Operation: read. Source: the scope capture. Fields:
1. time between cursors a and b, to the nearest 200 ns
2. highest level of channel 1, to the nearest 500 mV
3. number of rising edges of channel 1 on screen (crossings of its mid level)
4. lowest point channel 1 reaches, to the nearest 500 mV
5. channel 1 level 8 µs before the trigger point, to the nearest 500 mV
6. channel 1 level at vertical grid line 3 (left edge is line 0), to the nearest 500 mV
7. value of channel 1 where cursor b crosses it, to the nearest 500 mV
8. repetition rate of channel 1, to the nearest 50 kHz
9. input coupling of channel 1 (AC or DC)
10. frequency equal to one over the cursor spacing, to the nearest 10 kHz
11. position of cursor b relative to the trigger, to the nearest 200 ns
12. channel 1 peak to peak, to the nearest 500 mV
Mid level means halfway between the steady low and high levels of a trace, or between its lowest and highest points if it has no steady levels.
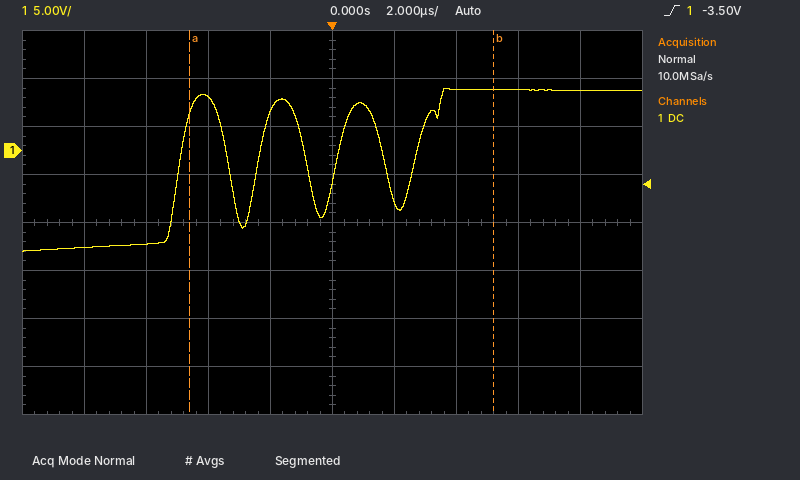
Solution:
9.8 µs
6.5 V
4
-10.5 V
-10.0 V
5.5 V
6.5 V
400 kHz
DC
100 kHz
+5.2 µs
17.0 V
